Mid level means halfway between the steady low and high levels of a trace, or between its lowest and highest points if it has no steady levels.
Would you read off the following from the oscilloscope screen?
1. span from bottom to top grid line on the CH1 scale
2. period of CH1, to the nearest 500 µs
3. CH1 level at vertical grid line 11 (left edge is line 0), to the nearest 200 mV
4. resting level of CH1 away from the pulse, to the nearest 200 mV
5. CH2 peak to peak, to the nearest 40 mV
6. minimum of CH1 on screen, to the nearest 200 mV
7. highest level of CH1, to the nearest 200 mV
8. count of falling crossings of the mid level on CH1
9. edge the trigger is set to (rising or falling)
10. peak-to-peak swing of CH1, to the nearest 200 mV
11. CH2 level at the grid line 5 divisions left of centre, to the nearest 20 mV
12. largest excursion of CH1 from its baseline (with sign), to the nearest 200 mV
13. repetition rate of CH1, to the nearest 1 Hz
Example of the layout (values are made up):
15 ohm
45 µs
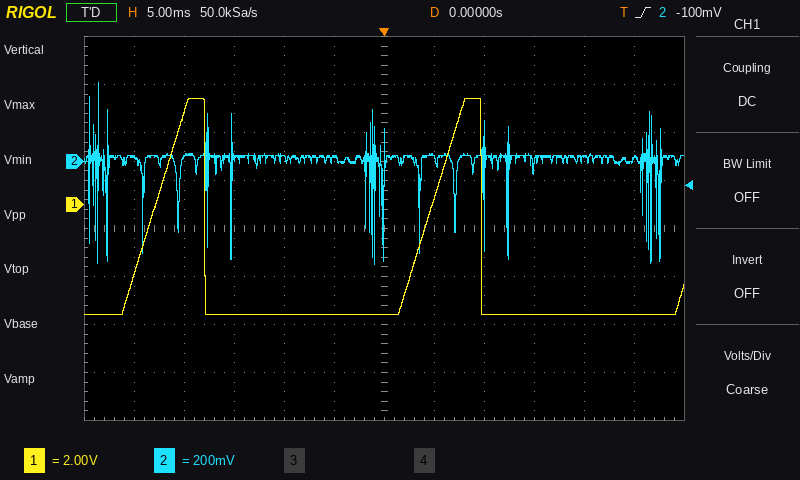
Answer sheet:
16 V
27.5 ms
-4.6 V
-4.6 V
760 mV
-4.6 V
4.4 V
2
rising
9.0 V
20 mV
+9.0 V
36 Hz
